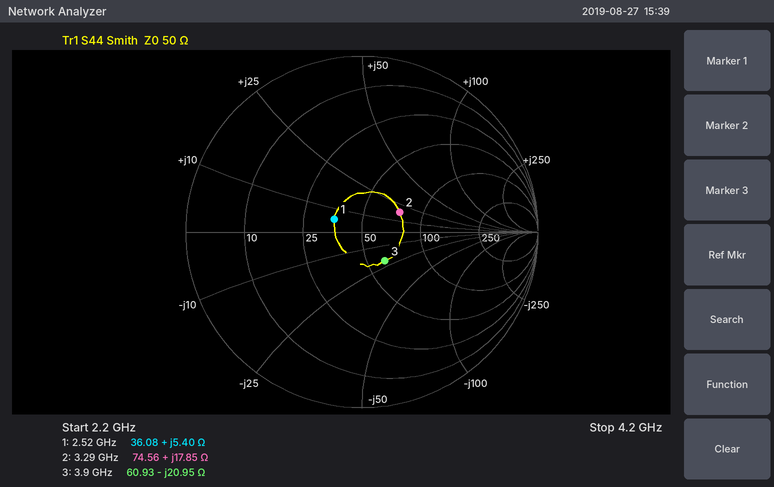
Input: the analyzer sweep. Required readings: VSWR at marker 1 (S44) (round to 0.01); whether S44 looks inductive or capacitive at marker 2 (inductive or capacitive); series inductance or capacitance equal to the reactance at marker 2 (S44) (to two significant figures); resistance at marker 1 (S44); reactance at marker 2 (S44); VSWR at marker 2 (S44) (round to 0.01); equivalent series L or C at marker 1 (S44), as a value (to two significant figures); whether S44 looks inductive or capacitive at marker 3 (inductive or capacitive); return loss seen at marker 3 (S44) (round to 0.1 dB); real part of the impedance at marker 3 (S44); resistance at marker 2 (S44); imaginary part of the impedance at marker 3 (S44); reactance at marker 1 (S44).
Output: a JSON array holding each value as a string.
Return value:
["1.42", "inductive", "860 pH", "36.08 Ω", "+17.85 Ω", "1.64", "340 pH", "capacitive", "13.6 dB", "60.93 Ω", "74.56 Ω", "-20.95 Ω", "+5.40 Ω"]
